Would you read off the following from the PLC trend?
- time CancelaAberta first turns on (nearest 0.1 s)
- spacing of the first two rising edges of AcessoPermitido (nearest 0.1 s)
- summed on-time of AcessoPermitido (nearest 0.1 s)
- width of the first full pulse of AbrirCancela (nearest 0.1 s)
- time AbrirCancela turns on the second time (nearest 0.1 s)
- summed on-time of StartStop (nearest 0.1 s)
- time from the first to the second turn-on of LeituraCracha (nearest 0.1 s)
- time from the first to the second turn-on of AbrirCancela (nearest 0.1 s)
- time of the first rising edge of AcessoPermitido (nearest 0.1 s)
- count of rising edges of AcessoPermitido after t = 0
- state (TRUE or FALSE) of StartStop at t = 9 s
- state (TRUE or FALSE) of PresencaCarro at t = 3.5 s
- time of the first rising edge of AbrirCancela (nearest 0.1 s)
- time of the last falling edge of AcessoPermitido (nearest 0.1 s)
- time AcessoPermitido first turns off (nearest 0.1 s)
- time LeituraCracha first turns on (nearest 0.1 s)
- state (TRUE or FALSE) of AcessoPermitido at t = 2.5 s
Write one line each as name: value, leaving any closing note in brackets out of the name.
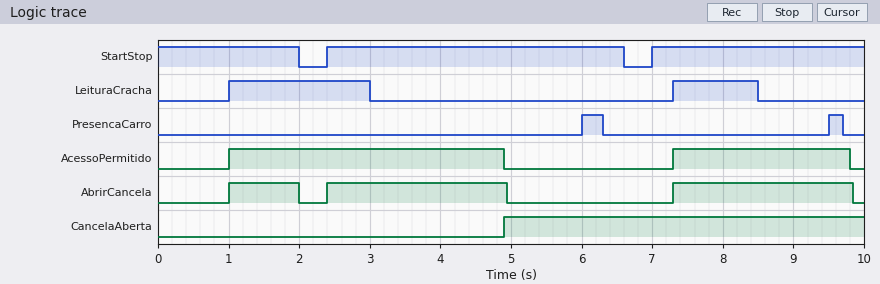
time CancelaAberta first turns on: 4.9 s
spacing of the first two rising edges of AcessoPermitido: 6.3 s
summed on-time of AcessoPermitido: 6.4 s
width of the first full pulse of AbrirCancela: 1.0 s
time AbrirCancela turns on the second time: 2.4 s
summed on-time of StartStop: 9.2 s
time from the first to the second turn-on of LeituraCracha: 6.3 s
time from the first to the second turn-on of AbrirCancela: 1.4 s
time of the first rising edge of AcessoPermitido: 1.0 s
count of rising edges of AcessoPermitido after t = 0: 2
state (TRUE or FALSE) of StartStop at t = 9 s: TRUE
state (TRUE or FALSE) of PresencaCarro at t = 3.5 s: FALSE
time of the first rising edge of AbrirCancela: 1.0 s
time of the last falling edge of AcessoPermitido: 9.8 s
time AcessoPermitido first turns off: 4.9 s
time LeituraCracha first turns on: 1.0 s
state (TRUE or FALSE) of AcessoPermitido at t = 2.5 s: TRUE
